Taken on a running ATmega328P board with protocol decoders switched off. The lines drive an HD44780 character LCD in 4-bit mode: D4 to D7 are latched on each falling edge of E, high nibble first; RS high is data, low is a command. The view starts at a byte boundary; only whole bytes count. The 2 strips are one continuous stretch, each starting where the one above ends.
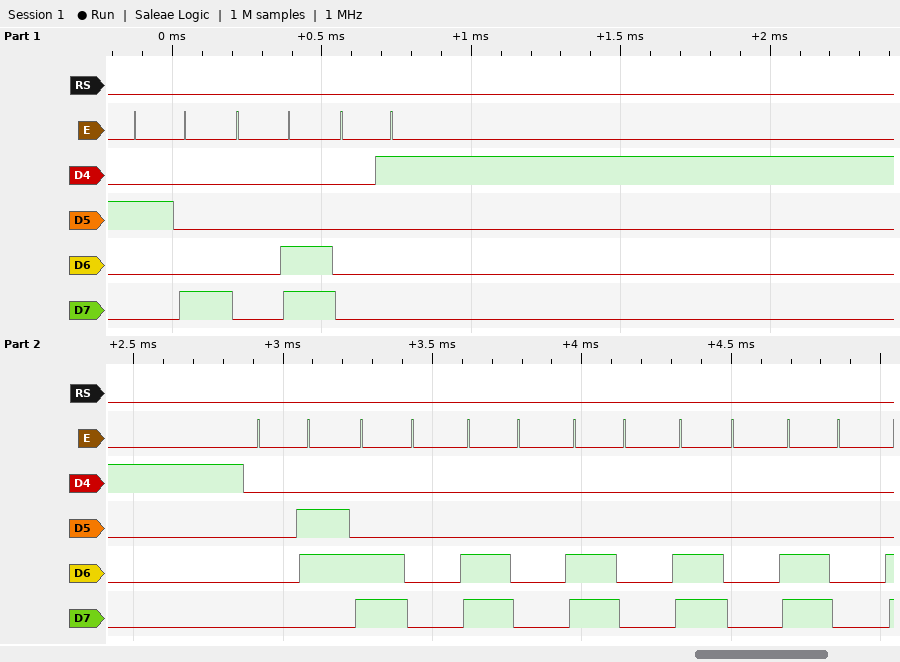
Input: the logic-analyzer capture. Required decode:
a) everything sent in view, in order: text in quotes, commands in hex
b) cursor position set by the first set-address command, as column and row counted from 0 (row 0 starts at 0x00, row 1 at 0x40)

0x28 0x0C 0x01 0x06 0xC0 0xC0 0xC0 0xC0 0xC0
column 0, row 1
